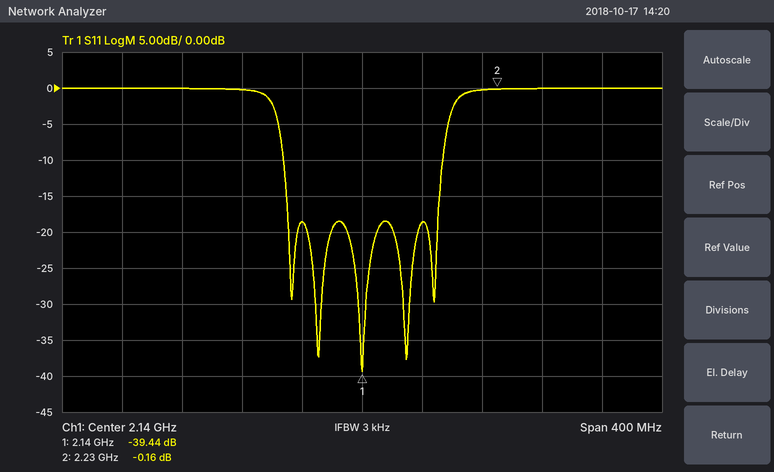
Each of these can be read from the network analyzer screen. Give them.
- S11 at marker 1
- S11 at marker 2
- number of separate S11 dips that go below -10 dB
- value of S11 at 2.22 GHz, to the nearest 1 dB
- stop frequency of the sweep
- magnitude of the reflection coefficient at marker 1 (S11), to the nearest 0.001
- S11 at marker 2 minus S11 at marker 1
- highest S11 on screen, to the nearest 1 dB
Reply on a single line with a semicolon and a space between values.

-39.44 dB; -0.16 dB; 5; 0 dB; 2.34 GHz; 0.011; 39.28 dB; 0 dB
